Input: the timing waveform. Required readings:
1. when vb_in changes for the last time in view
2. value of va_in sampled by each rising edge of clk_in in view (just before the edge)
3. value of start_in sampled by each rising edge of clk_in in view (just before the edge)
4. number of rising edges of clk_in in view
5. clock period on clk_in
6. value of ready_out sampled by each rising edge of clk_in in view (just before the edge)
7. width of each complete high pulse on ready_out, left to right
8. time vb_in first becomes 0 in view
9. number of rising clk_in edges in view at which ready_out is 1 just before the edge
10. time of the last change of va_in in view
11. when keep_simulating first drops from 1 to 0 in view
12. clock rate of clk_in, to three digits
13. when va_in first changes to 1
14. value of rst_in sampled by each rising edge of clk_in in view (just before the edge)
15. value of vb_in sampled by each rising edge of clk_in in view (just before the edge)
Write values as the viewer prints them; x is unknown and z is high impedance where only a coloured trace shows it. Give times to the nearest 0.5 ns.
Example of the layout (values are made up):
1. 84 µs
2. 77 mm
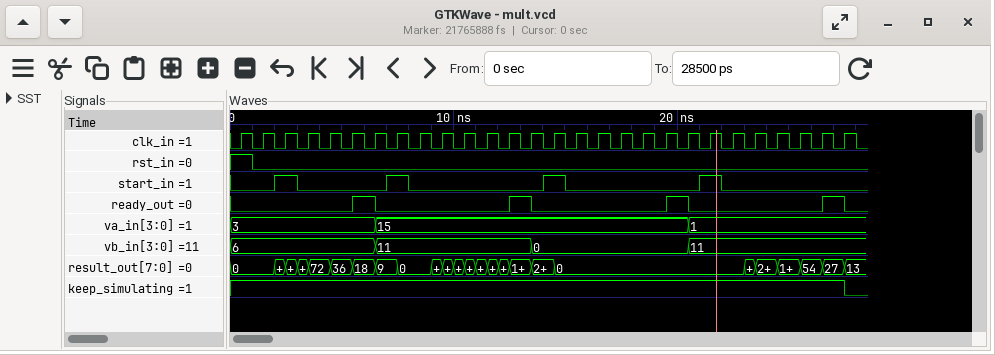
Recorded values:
1. 20.5 ns
2. 3, 3, 3, 3, 3, 3, 3, 15, 15, 15, 15, 15, 15, 15, 15, 15, 15, 15, 15, 15, 15, 1, 1, 1, 1, 1, 1, 1
3. 0 0 1 0 0 0 0 1 0 0 0 0 0 0 1 0 0 0 0 0 0 1 0 0 0 0 0 0
4. 28
5. 1 ns
6. 0 0 0 0 0 0 1 0 0 0 0 0 0 1 0 0 0 0 0 0 1 0 0 0 0 0 0 1
7. 1 ns, 1 ns, 1 ns, 1 ns
8. 13.5 ns
9. 4
10. 20.5 ns
11. 27.5 ns
12. 1.00 GHz
13. 20.5 ns
14. 1 0 0 0 0 0 0 0 0 0 0 0 0 0 0 0 0 0 0 0 0 0 0 0 0 0 0 0
15. 6, 6, 6, 6, 6, 6, 6, 11, 11, 11, 11, 11, 11, 11, 0, 0, 0, 0, 0, 0, 0, 11, 11, 11, 11, 11, 11, 11
